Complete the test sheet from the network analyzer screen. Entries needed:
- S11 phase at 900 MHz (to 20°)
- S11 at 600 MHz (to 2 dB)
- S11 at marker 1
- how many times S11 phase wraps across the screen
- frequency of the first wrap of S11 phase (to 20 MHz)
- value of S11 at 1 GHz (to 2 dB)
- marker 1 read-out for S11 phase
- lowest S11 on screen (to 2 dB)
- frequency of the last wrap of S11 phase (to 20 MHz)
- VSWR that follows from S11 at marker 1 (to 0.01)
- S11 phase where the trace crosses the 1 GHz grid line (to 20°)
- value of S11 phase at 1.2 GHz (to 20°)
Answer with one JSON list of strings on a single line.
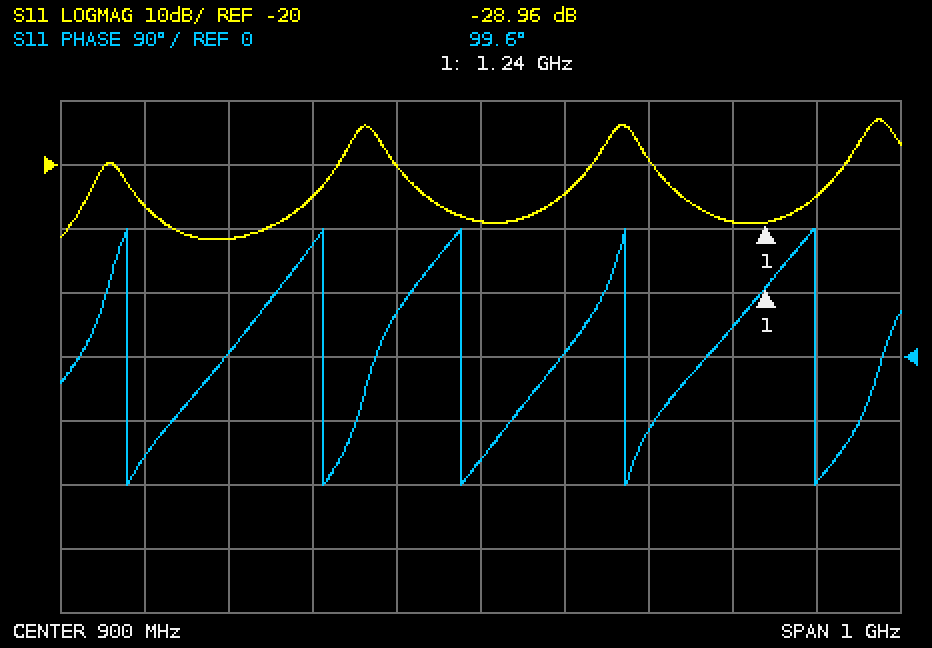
["-140°", "-32 dB", "-28.96 dB", "5", "480 MHz", "-24 dB", "99.6°", "-32 dB", "1.30 GHz", "1.07", "0°", "40°"]
